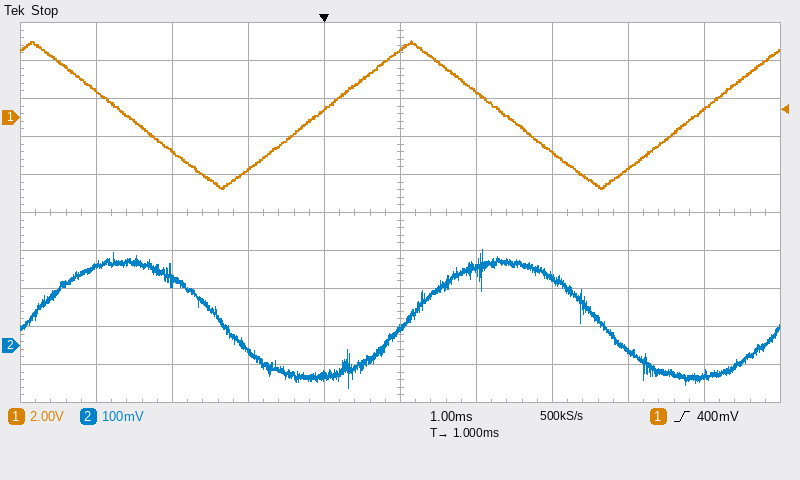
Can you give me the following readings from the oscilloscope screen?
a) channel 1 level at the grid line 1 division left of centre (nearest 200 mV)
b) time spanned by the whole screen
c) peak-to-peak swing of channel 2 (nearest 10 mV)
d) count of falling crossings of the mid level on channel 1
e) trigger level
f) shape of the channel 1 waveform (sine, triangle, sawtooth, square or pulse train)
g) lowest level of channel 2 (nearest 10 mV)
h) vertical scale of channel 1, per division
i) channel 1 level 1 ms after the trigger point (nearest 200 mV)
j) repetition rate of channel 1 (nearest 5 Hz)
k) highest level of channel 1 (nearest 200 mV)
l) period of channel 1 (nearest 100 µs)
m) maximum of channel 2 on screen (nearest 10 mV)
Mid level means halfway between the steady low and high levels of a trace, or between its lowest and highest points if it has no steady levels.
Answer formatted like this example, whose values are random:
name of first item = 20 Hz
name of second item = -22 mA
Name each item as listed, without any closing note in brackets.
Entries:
channel 1 level at the grid line 1 division left of centre = 400 mV
time spanned by the whole screen = 10 ms
peak-to-peak swing of channel 2 = 360 mV
count of falling crossings of the mid level on channel 1 = 2
trigger level = 400 mV
shape of the channel 1 waveform = triangle
lowest level of channel 2 = -110 mV
vertical scale of channel 1, per division = 2 V
channel 1 level 1 ms after the trigger point = 3.6 V
repetition rate of channel 1 = 200 Hz
highest level of channel 1 = 4.0 V
period of channel 1 = 5.0 ms
maximum of channel 2 on screen = 250 mV
